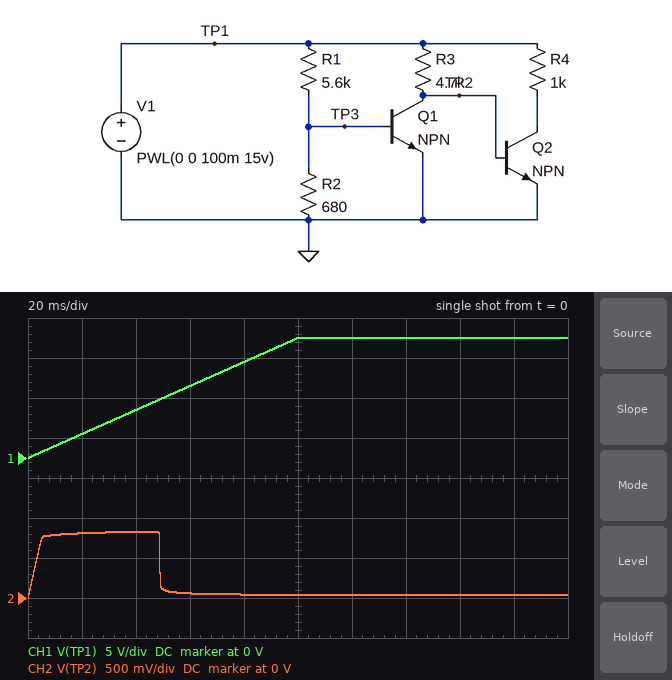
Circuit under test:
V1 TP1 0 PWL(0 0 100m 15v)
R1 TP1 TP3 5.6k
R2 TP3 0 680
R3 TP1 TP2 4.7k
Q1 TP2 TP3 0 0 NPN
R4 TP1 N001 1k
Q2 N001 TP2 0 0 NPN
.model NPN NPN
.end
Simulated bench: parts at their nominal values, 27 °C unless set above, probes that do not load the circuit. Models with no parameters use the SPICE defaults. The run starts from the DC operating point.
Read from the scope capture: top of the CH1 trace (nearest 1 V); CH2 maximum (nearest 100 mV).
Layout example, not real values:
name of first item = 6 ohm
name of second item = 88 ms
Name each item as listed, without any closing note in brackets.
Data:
top of the CH1 trace = 15 V
CH2 maximum = 800 mV
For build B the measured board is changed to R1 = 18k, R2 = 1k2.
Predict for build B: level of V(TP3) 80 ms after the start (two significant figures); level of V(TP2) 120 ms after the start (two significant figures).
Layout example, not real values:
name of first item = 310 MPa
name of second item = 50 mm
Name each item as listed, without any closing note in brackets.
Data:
level of V(TP3) 80 ms after the start = 750 mV
level of V(TP2) 120 ms after the start = 95 mV
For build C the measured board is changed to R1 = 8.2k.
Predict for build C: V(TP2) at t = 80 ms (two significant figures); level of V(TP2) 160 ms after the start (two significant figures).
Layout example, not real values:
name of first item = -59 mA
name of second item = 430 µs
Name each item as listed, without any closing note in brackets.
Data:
V(TP2) at t = 80 ms = 75 mV
level of V(TP2) 160 ms after the start = 55 mV
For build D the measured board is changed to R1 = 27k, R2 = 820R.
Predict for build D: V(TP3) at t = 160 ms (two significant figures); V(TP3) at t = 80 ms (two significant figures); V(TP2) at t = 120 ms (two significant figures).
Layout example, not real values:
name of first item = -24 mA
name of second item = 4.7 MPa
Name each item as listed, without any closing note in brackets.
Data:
V(TP3) at t = 160 ms = 440 mV
V(TP3) at t = 80 ms = 350 mV
V(TP2) at t = 120 ms = 850 mV
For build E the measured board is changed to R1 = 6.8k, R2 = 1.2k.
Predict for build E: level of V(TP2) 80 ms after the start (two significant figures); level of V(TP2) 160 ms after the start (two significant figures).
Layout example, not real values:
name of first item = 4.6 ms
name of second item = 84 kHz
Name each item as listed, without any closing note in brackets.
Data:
level of V(TP2) 80 ms after the start = 40 mV
level of V(TP2) 160 ms after the start = 38 mV
